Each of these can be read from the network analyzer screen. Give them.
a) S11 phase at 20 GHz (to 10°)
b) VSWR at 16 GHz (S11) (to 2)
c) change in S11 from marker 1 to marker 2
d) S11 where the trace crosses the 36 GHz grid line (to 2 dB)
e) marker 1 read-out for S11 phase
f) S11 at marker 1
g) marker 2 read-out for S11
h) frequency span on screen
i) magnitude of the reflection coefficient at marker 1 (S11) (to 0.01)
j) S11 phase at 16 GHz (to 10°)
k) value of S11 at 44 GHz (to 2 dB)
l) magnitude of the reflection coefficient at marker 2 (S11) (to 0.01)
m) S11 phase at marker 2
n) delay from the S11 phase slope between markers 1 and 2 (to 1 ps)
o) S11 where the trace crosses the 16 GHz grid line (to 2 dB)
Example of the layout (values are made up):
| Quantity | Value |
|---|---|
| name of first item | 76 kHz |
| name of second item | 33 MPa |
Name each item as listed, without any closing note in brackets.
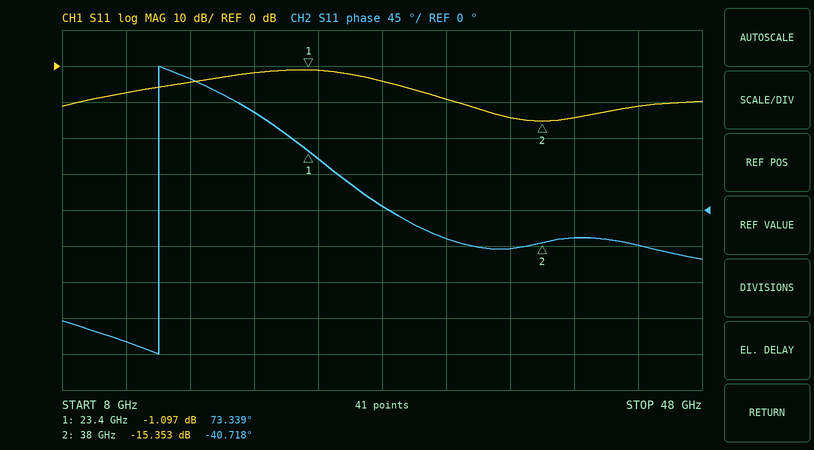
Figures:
| Quantity | Value |
|---|---|
| S11 phase at 20 GHz | 120° |
| VSWR at 16 GHz (S11) | 4 |
| change in S11 from marker 1 to marker 2 | -14.256 dB |
| S11 where the trace crosses the 36 GHz grid line | -14 dB |
| marker 1 read-out for S11 phase | 73.339° |
| S11 at marker 1 | -1.097 dB |
| marker 2 read-out for S11 | -15.353 dB |
| frequency span on screen | 40 GHz |
| magnitude of the reflection coefficient at marker 1 (S11) | 0.88 |
| S11 phase at 16 GHz | 160° |
| value of S11 at 44 GHz | -12 dB |
| magnitude of the reflection coefficient at marker 2 (S11) | 0.17 |
| S11 phase at marker 2 | -40.718° |
| delay from the S11 phase slope between markers 1 and 2 | 22 ps |
| S11 where the trace crosses the 16 GHz grid line | -4 dB |
